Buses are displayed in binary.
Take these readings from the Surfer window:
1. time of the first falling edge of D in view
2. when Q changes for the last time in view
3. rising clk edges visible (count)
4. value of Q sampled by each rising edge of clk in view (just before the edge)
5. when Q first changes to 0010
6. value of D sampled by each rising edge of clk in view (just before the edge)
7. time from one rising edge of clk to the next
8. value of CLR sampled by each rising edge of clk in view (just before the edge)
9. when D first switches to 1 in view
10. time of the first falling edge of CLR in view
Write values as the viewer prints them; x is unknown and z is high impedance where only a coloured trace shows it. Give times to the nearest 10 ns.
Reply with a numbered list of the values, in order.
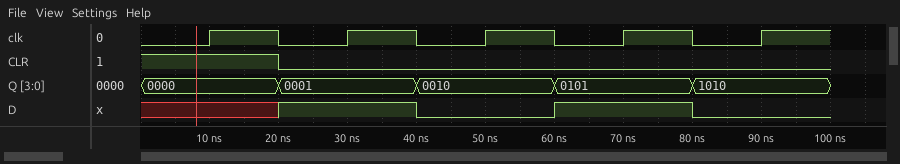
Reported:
1. 40 ns
2. 80 ns
3. 5
4. 0000, 0001, 0010, 0101, 1010
5. 40 ns
6. x 1 0 1 0
7. 20 ns
8. 1 0 0 0 0
9. 20 ns
10. 20 ns
